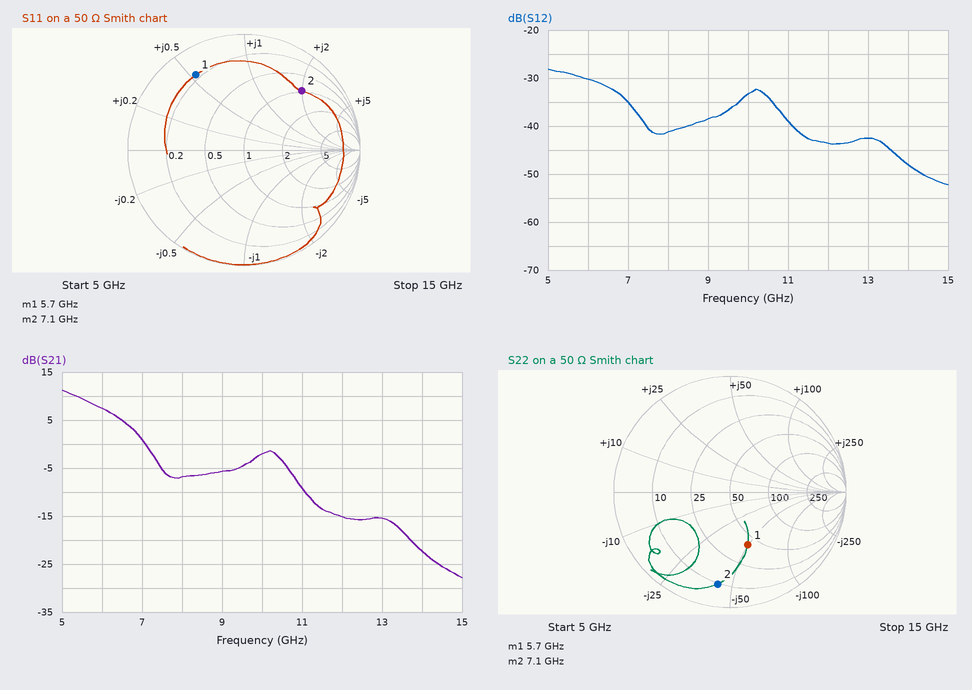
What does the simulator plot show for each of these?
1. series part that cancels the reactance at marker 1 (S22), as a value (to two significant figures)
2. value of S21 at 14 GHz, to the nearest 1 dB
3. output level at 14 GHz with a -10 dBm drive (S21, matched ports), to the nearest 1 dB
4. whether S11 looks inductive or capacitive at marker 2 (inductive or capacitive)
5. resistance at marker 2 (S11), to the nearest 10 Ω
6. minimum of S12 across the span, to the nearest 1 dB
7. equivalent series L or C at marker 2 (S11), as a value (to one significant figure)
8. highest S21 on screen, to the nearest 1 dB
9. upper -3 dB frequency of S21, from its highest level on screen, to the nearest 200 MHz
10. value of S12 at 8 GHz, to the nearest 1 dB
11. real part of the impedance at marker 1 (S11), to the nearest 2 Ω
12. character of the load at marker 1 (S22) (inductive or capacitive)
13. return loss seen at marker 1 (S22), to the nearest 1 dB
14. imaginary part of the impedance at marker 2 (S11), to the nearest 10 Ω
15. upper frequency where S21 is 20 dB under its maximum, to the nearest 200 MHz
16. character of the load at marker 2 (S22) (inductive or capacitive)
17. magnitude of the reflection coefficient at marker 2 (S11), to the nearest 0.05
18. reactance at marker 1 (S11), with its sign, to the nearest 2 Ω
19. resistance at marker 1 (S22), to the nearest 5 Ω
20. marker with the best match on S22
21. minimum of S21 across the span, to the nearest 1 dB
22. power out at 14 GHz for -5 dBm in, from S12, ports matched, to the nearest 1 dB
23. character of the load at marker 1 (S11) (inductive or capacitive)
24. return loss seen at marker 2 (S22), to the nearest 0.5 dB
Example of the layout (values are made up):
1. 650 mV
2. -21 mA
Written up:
1. 1.4 nH
2. -22 dB
3. -32 dBm
4. inductive
5. 50 Ω
6. -52 dB
7. 2 nH
8. 11 dB
9. 5.8 GHz
10. -41 dB
11. 8 Ω
12. capacitive
13. 6 dB
14. +100 Ω
15. 11.0 GHz
16. capacitive
17. 0.70
18. +26 Ω
19. 40 Ω
20. marker 1
21. -28 dB
22. -53 dBm
23. inductive
24. 2.0 dB
